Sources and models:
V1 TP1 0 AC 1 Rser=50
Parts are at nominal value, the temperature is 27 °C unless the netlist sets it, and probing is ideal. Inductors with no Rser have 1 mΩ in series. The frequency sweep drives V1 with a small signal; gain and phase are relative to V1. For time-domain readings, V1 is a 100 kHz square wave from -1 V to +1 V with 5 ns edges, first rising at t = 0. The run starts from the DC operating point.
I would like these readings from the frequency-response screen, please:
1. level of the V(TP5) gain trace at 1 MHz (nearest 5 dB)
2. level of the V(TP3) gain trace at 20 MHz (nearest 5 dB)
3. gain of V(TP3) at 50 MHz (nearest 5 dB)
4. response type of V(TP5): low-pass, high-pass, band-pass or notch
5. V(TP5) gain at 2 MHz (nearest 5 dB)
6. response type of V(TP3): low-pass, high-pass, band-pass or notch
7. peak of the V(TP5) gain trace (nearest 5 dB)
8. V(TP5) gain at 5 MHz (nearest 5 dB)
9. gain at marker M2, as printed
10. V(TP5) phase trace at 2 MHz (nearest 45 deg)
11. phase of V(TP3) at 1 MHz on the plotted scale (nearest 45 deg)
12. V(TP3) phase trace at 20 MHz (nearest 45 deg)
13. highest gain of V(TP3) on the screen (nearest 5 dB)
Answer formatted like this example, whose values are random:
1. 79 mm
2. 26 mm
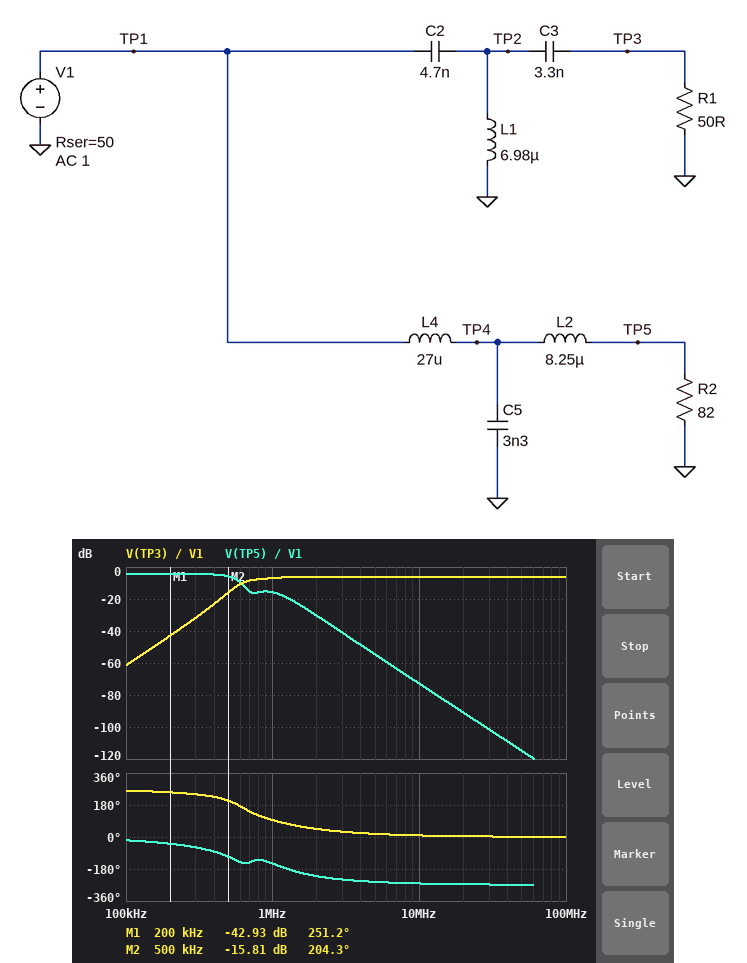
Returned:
1. -15 dB
2. -5 dB
3. -5 dB
4. low-pass
5. -30 dB
6. high-pass
7. -5 dB
8. -55 dB
9. -15.81 dB
10. -225 deg
11. 90 deg
12. 0 deg
13. -5 dB
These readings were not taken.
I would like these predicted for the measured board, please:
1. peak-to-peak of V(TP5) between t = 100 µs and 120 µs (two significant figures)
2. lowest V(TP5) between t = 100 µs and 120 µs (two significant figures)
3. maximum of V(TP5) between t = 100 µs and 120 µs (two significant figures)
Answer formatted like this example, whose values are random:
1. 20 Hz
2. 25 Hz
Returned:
1. 1.5 V
2. -740 mV
3. 740 mV
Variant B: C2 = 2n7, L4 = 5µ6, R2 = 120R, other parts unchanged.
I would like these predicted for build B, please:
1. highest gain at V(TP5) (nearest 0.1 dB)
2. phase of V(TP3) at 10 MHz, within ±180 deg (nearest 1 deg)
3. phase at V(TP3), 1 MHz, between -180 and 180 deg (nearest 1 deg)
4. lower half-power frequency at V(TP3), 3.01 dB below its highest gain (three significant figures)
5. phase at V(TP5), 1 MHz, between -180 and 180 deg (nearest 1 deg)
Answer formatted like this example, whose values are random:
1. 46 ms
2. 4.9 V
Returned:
1. -3.0 dB
2. 14 deg
3. 90 deg
4. 1.72 MHz
5. -79 deg
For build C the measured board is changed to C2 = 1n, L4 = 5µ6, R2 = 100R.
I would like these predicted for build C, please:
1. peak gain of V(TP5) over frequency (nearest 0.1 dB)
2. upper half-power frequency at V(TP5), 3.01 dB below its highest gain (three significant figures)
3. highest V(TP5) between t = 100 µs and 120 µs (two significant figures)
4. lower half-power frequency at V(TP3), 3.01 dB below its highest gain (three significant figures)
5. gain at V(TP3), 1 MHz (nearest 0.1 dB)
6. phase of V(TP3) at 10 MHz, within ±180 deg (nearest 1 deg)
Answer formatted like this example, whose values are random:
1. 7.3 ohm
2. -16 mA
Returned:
1. -3.5 dB
2. 1.54 MHz
3. 740 mV
4. 1.93 MHz
5. -18.3 dB
6. 19 deg
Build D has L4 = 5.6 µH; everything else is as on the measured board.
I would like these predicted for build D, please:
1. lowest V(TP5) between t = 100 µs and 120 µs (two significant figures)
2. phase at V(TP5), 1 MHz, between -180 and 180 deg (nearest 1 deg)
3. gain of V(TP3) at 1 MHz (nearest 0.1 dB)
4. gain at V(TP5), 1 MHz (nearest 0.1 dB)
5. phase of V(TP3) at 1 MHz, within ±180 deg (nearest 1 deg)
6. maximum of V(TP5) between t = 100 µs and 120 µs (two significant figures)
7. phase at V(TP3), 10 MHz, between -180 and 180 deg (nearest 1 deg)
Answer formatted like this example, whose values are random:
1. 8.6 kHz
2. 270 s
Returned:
1. -730 mV
2. -71 deg
3. -10.4 dB
4. -7.5 dB
5. 71 deg
6. 730 mV
7. 12 deg
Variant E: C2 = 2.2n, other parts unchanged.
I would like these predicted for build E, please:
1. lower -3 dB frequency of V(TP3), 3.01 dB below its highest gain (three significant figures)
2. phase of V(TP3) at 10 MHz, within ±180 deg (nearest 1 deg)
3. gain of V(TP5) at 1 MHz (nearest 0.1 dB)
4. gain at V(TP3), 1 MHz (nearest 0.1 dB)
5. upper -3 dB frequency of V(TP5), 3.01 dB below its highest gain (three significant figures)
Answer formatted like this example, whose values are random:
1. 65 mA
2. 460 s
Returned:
1. 782 kHz
2. 11 deg
3. -14.3 dB
4. -6.5 dB
5. 745 kHz
